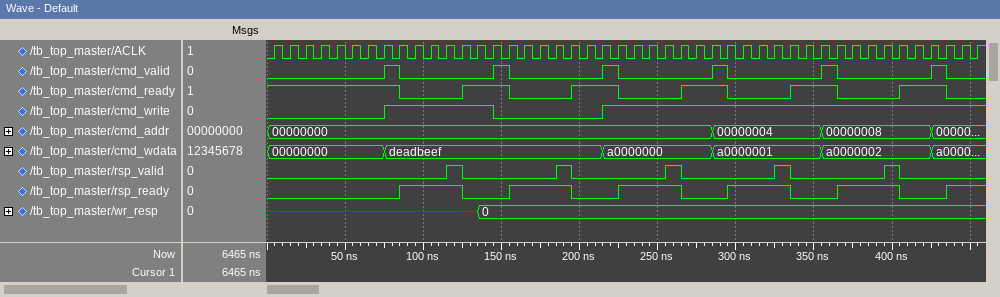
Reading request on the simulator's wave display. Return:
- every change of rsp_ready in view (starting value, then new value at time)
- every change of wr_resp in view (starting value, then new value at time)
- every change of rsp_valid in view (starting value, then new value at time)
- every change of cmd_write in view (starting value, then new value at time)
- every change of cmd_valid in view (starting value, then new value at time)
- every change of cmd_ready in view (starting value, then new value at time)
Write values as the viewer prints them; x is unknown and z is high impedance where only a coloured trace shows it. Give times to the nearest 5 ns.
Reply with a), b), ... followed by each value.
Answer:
a) 0, 1 at 85 ns, 0 at 125 ns, 1 at 155 ns, 0 at 195 ns, 1 at 225 ns, 0 at 265 ns, 1 at 295 ns, 0 at 335 ns, 1 at 365 ns, 0 at 405 ns, 1 at 435 ns
b) x, 0 at 135 ns
c) 0, 1 at 115 ns, 0 at 125 ns, 1 at 185 ns, 0 at 195 ns, 1 at 255 ns, 0 at 265 ns, 1 at 325 ns, 0 at 335 ns, 1 at 395 ns, 0 at 405 ns
d) 0, 1 at 75 ns, 0 at 145 ns, 1 at 215 ns
e) 0, 1 at 75 ns, 0 at 85 ns, 1 at 145 ns, 0 at 155 ns, 1 at 215 ns, 0 at 225 ns, 1 at 285 ns, 0 at 295 ns, 1 at 355 ns, 0 at 365 ns, 1 at 425 ns, 0 at 435 ns
f) 1, 0 at 85 ns, 1 at 125 ns, 0 at 155 ns, 1 at 195 ns, 0 at 225 ns, 1 at 265 ns, 0 at 295 ns, 1 at 335 ns, 0 at 365 ns, 1 at 405 ns, 0 at 435 ns
